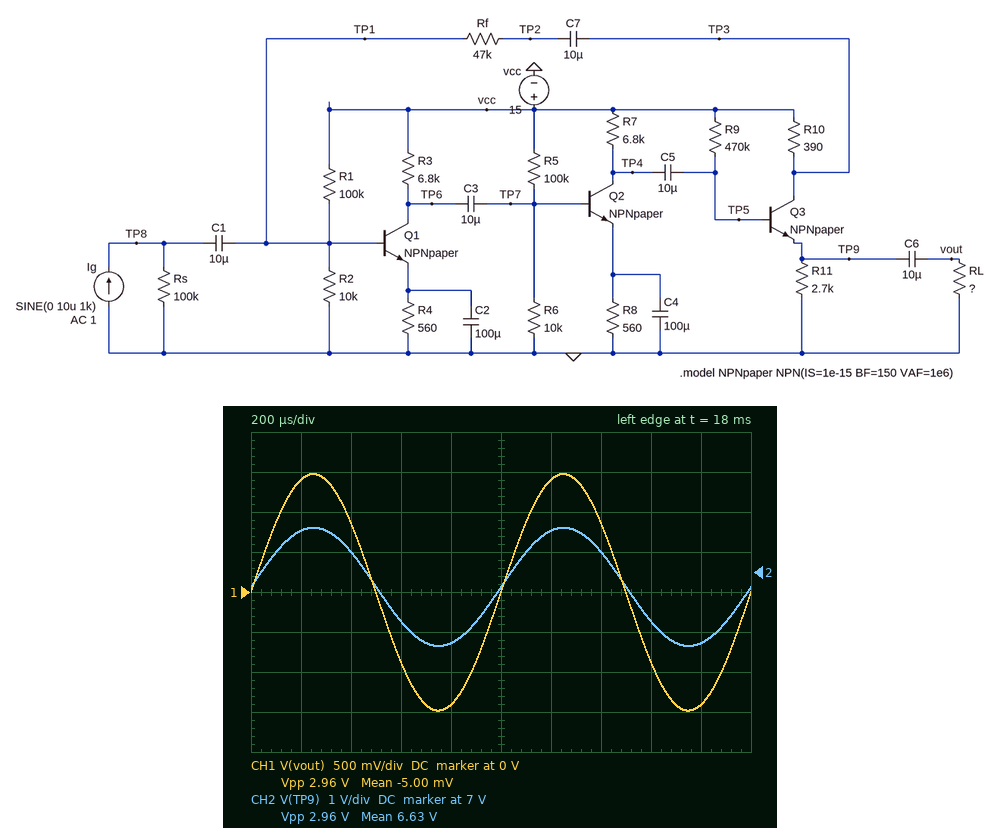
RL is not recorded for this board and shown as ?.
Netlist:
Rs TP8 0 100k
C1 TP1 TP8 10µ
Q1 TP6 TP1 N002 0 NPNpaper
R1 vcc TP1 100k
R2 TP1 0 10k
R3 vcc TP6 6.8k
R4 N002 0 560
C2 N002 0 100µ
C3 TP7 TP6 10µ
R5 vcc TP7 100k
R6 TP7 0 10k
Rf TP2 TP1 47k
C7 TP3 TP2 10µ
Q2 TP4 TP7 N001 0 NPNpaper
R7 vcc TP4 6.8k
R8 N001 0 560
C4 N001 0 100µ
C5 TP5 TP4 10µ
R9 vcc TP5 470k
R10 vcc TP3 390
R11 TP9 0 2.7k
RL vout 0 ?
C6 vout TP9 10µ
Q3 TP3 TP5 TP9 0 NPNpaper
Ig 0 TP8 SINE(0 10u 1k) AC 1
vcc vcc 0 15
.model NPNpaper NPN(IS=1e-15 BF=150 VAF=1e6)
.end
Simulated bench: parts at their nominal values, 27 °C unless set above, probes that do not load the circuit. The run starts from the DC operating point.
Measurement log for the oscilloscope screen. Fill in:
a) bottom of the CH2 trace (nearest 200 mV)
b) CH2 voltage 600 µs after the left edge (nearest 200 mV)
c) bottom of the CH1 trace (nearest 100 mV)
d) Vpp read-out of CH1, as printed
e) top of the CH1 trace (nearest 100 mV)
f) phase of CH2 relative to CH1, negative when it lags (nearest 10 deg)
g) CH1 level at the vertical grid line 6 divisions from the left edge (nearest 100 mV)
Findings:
5.2 V
5.8 V
-1.5 V
2.96 V
1.5 V
0 deg
1.4 V
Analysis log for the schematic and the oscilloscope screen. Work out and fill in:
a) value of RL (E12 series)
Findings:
2.2 kΩ
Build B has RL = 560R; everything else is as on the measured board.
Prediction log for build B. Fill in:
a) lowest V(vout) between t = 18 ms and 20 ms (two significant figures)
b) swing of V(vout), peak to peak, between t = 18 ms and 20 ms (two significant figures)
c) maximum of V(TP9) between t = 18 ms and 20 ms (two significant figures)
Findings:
-570 mV
1.1 V
7.2 V
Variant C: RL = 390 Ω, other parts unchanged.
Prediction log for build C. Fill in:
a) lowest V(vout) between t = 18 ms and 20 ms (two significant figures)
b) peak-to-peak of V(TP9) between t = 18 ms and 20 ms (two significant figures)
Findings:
-420 mV
830 mV
